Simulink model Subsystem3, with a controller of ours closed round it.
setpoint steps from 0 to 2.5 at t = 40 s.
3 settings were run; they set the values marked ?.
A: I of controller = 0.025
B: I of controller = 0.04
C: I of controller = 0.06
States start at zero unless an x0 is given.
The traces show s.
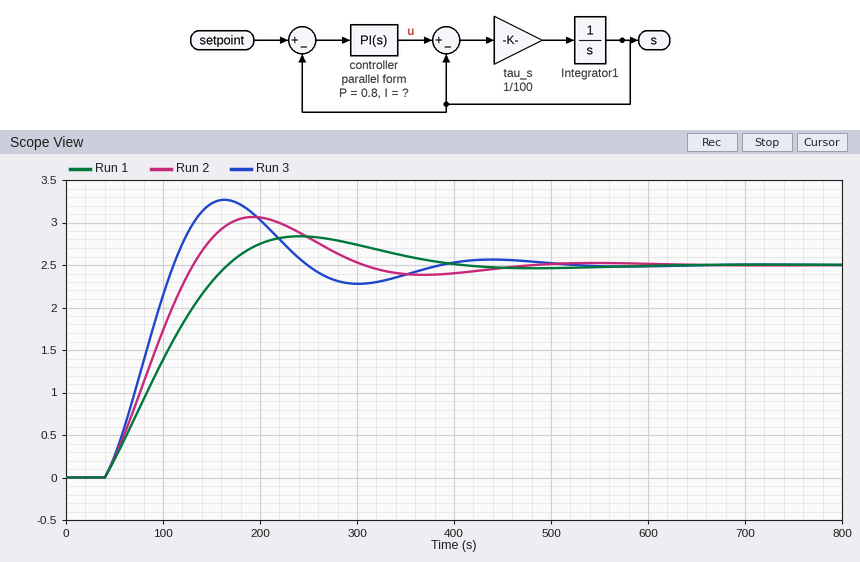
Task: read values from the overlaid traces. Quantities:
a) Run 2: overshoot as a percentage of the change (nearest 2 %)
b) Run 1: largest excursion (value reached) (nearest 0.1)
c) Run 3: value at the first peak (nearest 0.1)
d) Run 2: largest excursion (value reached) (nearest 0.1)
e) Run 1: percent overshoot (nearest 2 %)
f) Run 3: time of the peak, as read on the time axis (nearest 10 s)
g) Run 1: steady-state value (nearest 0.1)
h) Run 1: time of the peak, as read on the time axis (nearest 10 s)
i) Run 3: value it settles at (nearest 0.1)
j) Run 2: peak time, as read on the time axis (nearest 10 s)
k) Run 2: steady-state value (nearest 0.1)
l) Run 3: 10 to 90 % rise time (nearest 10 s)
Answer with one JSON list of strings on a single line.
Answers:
["22 %", "2.8", "3.3", "3.1", "14 %", "160 s", "2.5", "240 s", "2.5", "190 s", "2.5", "50 s"]
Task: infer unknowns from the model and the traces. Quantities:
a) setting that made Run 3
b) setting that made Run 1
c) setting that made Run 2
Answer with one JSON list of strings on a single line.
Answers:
["C", "A", "B"]
